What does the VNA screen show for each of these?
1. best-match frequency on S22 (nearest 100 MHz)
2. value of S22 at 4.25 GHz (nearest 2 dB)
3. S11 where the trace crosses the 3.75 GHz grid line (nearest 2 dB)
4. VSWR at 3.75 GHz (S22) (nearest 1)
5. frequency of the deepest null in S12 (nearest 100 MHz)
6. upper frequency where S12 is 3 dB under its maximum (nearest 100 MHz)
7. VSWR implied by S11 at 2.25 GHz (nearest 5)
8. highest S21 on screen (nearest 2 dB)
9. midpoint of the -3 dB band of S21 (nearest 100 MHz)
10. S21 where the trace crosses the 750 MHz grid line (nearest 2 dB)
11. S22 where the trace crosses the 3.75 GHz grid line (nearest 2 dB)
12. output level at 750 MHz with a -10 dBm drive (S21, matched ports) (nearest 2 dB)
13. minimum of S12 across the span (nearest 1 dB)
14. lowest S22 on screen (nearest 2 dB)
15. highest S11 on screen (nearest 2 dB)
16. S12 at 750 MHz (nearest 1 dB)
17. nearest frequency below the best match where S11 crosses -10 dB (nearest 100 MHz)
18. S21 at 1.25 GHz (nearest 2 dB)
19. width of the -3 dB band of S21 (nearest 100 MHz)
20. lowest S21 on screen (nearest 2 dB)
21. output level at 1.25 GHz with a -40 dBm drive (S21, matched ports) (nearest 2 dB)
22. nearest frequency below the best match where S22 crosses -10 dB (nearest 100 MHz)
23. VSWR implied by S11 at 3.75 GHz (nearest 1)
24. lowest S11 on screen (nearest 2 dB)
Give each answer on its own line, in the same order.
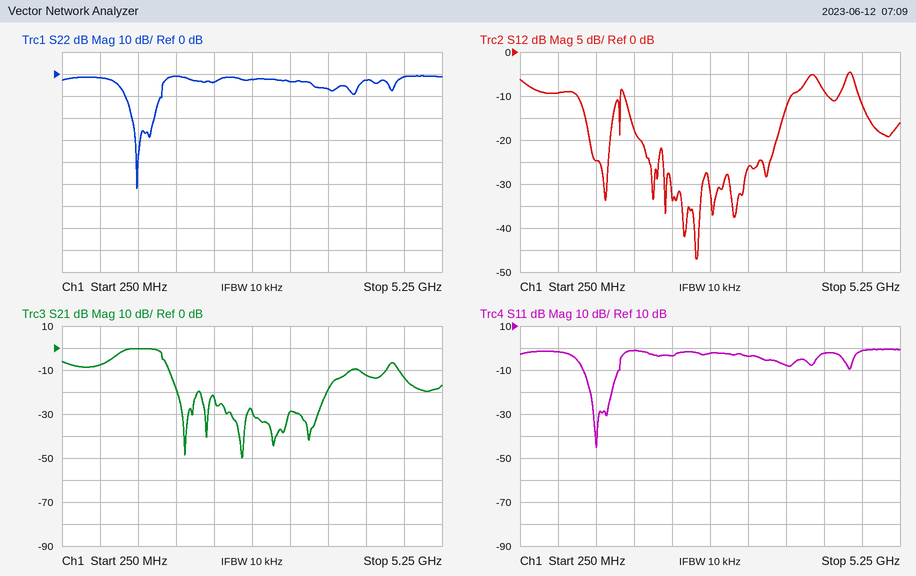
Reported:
1.2 GHz
-2 dB
-8 dB
3
2.6 GHz
4.7 GHz
5
0 dB
1.3 GHz
-8 dB
-6 dB
-18 dBm
-47 dB
-52 dB
0 dB
-9 dB
1.1 GHz
0 dB
600 MHz
-50 dB
-40 dBm
1.1 GHz
2
-46 dB
